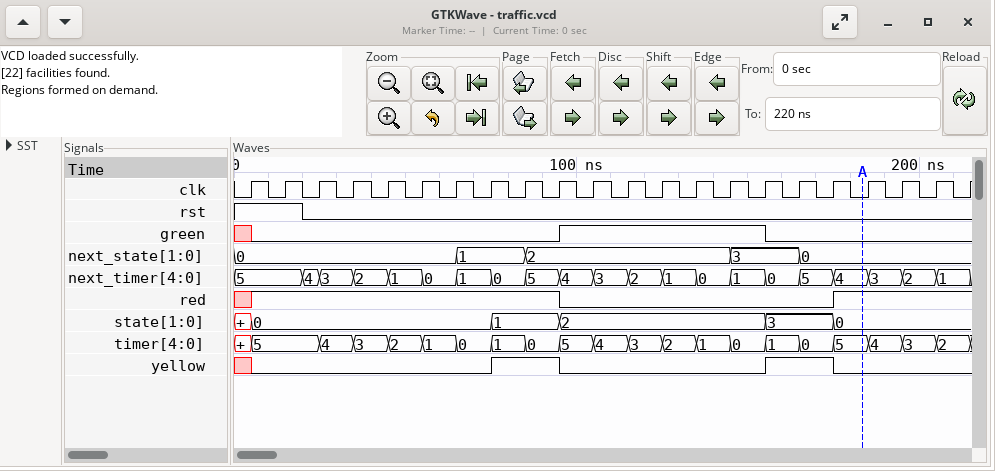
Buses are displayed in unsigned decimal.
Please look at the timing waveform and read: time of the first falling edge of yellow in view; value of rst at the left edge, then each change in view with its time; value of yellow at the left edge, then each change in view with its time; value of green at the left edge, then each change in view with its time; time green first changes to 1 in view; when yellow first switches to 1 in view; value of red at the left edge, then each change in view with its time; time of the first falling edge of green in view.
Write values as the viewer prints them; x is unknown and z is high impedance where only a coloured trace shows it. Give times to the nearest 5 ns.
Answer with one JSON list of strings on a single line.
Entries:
["95 ns", "1, 0 at 20 ns", "x, 0 at 5 ns, 1 at 75 ns, 0 at 95 ns, 1 at 155 ns, 0 at 175 ns", "x, 0 at 5 ns, 1 at 95 ns, 0 at 155 ns", "95 ns", "75 ns", "x, 1 at 5 ns, 0 at 95 ns, 1 at 175 ns", "155 ns"]
